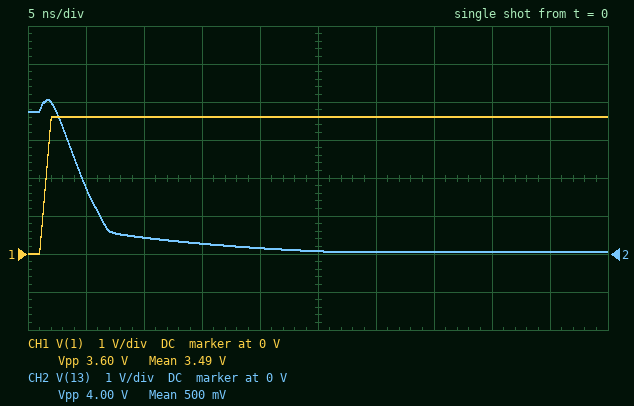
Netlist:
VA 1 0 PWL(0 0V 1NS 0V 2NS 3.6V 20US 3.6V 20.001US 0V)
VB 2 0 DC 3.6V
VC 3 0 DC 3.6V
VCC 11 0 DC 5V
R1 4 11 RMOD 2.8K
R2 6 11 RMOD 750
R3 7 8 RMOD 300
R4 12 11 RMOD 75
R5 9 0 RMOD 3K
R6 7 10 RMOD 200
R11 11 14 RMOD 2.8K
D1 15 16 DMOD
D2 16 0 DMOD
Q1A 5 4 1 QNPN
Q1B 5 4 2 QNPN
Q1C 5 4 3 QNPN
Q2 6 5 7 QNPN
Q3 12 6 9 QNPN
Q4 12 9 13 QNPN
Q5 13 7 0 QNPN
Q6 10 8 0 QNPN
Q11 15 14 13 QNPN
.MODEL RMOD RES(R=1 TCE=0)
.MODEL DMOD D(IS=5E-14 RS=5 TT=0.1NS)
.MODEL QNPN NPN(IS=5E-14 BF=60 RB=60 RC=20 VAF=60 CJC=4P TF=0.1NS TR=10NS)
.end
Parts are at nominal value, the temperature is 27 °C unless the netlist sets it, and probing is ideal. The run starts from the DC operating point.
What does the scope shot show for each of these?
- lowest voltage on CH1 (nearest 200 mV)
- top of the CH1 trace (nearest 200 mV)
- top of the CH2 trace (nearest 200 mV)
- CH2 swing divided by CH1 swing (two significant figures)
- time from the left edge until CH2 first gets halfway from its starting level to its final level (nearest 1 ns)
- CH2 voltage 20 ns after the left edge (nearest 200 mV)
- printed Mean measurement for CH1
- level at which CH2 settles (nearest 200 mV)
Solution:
0 V
3.6 V
4.0 V
1.1
5 ns
200 mV
3.49 V
0 V
